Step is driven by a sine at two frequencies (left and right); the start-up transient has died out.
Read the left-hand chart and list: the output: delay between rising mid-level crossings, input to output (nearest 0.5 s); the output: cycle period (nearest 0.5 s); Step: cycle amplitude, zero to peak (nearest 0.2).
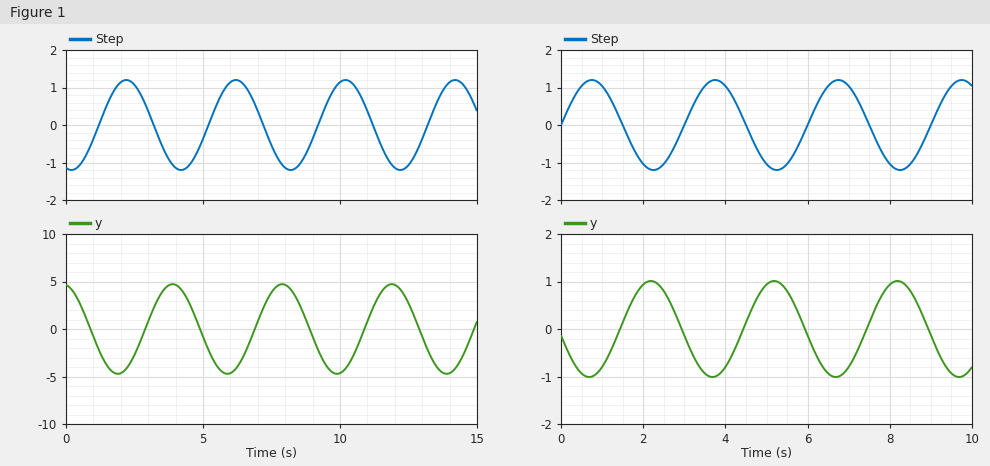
1.5 s
4.0 s
1.2
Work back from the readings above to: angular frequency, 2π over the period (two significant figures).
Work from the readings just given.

1.6 rad/s
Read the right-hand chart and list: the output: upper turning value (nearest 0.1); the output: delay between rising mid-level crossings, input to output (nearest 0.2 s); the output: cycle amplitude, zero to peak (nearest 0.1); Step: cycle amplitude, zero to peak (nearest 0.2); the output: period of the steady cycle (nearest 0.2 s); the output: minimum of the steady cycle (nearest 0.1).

1.0
1.4 s
1.0
1.2
3.0 s
-1.0
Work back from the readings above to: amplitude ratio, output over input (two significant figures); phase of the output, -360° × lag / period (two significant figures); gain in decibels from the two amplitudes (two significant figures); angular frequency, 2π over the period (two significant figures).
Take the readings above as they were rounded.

0.83
-170°
-1.6 dB
2.1 rad/s
